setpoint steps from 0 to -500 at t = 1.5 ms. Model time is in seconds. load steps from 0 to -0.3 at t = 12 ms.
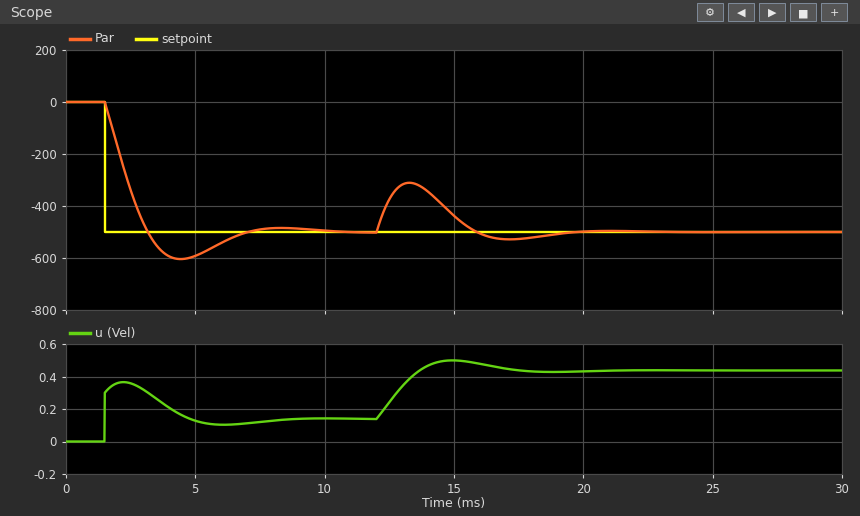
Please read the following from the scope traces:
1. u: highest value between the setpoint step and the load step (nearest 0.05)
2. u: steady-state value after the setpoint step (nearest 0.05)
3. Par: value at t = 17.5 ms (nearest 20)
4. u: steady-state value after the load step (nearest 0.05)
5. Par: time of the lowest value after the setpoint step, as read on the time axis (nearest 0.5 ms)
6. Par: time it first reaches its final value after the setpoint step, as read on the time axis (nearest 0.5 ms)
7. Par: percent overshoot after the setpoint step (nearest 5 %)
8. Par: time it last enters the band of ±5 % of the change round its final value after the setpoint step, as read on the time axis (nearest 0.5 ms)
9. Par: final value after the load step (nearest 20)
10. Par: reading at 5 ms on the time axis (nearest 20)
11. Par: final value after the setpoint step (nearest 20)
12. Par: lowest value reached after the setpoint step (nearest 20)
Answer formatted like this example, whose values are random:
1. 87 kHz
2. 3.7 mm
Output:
1. 0.35
2. 0.15
3. -520
4. 0.45
5. 4.5 ms
6. 3.0 ms
7. 20 %
8. 6.5 ms
9. -500
10. -600
11. -500
12. -600
